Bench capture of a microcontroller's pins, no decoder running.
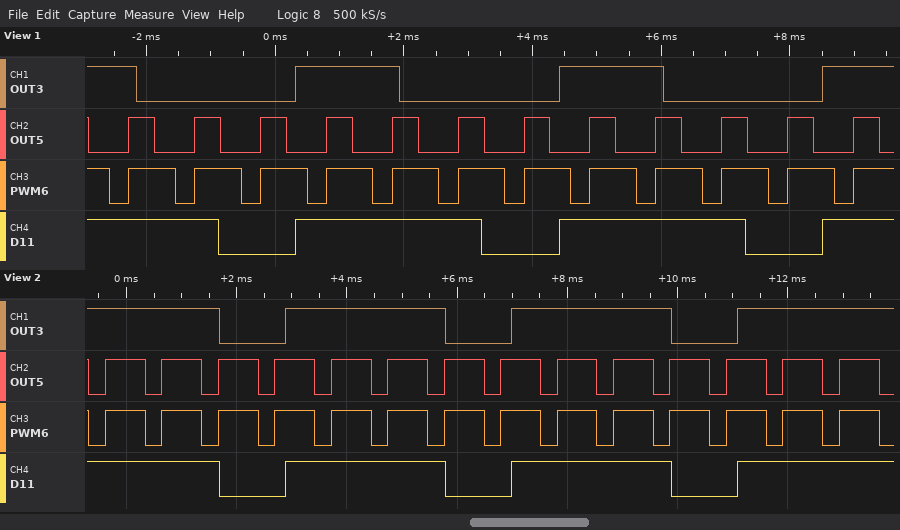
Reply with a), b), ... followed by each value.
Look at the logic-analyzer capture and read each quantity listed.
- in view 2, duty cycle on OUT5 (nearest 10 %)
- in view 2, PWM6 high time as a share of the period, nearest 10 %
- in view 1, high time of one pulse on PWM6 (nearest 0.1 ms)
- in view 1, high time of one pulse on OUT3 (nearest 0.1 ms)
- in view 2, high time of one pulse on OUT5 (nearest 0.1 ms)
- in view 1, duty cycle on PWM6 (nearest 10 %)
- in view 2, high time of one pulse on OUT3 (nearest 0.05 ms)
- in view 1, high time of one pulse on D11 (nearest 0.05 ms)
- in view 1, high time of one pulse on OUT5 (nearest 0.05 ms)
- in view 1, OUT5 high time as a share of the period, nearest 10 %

a) 70 %
b) 70 %
c) 0.7 ms
d) 1.6 ms
e) 0.7 ms
f) 70 %
g) 2.90 ms
h) 2.90 ms
i) 0.40 ms
j) 40 %
